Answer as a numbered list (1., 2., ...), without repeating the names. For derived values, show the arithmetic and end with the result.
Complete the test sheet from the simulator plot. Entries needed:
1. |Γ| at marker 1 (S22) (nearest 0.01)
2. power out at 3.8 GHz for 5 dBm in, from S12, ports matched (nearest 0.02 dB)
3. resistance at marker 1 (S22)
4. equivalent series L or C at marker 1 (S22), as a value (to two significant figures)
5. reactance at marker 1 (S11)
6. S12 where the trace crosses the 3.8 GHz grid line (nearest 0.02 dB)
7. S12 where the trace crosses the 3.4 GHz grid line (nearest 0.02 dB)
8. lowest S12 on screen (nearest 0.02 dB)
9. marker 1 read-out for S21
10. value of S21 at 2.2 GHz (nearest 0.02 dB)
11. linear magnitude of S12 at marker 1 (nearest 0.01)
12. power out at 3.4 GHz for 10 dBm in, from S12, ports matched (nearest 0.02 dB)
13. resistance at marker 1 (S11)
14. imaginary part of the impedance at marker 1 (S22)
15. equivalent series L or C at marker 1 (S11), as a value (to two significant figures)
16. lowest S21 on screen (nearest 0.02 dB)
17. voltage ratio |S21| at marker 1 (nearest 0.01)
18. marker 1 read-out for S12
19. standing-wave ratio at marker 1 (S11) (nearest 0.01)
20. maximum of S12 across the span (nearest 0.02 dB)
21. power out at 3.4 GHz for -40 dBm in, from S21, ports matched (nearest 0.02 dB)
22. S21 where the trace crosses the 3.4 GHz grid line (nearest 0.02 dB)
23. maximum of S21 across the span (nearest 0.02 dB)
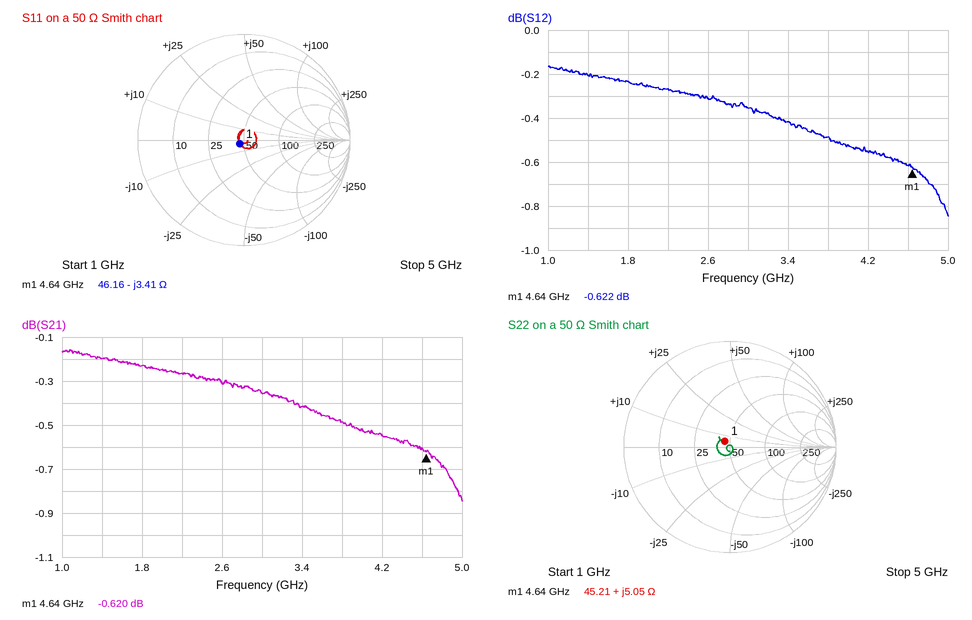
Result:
1. 0.07
2. 5 dBm + (-0.48 dB) = 4.52 dBm
3. 45.21 Ω
4. L = 5.05 Ω/(2π × 4.64 GHz) ≈ 173 pH, so 170 pH to two significant figures
5. -3.41 Ω
6. -0.48 dB
7. -0.42 dB
8. -0.84 dB
9. -0.620 dB
10. -0.26 dB
11. 10^(-0.622/20) ≈ 0.93
12. 10 dBm + (-0.42 dB) = 9.58 dBm
13. 46.16 Ω
14. +5.05 Ω
15. C = 1/(2π × 4.64 GHz × 3.41 Ω) ≈ 10 pF
16. -0.84 dB
17. 10^(-0.62/20) ≈ 0.93
18. -0.622 dB
19. 1.11
20. -0.16 dB
21. -40 dBm + (-0.42 dB) = -40.42 dBm
22. -0.42 dB
23. -0.16 dB
